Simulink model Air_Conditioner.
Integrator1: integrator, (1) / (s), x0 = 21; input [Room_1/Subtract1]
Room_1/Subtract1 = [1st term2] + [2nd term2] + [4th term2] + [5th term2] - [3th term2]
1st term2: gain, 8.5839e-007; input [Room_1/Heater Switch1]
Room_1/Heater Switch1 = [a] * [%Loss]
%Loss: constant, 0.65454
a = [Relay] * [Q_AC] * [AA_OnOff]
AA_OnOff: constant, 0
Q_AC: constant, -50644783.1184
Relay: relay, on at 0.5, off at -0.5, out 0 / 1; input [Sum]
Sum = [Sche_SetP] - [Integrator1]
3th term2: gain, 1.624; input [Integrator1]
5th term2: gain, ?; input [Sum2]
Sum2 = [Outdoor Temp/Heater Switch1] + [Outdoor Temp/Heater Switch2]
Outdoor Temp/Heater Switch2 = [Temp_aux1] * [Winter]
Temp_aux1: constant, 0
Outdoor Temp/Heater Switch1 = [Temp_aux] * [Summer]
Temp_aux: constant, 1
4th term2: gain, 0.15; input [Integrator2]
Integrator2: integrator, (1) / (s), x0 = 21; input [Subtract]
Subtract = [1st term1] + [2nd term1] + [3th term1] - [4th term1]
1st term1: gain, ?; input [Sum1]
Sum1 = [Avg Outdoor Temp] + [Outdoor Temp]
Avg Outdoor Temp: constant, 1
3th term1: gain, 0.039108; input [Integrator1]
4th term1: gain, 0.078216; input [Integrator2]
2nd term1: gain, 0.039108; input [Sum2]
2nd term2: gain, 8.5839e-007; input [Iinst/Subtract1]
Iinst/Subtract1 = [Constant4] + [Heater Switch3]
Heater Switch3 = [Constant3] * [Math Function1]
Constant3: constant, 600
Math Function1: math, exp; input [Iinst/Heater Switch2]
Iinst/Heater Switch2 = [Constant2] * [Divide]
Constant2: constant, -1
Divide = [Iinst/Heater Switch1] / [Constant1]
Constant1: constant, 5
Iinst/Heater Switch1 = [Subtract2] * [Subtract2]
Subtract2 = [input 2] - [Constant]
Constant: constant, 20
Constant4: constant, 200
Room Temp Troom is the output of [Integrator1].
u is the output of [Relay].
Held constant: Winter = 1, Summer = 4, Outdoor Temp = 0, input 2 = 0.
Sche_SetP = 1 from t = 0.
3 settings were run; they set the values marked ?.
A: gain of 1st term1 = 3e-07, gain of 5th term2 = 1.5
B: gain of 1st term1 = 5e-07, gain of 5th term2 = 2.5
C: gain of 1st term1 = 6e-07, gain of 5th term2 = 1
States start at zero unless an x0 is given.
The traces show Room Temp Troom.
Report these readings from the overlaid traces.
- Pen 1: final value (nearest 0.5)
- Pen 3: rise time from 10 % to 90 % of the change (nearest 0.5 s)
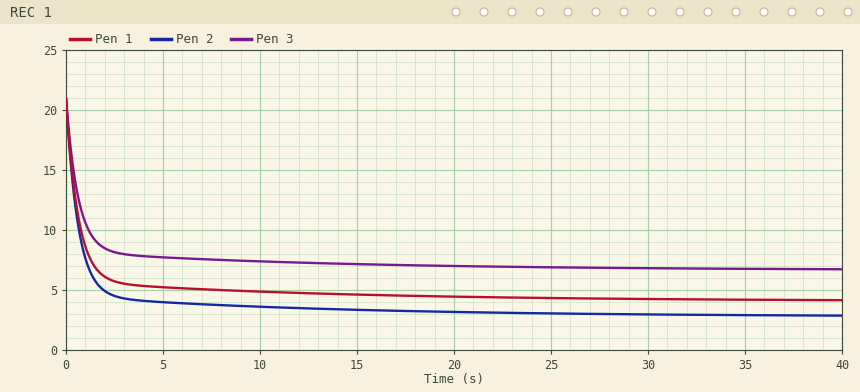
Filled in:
4.0
2.5 s
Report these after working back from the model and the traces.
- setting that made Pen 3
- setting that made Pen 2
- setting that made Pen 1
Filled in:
B
C
A
